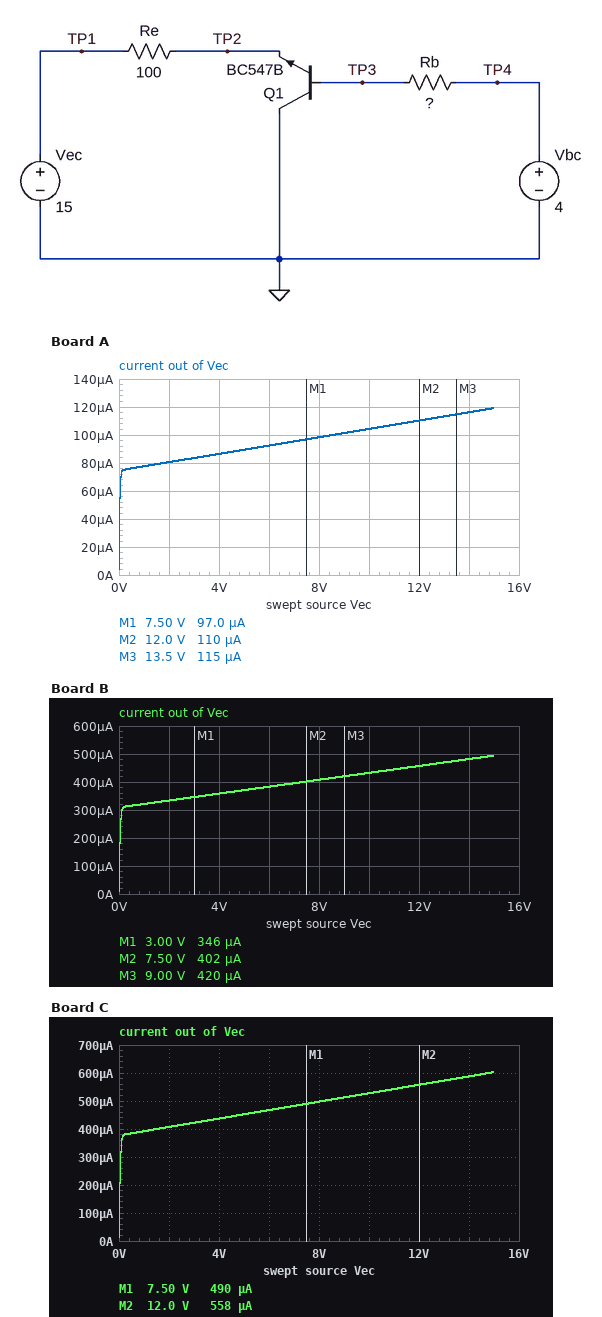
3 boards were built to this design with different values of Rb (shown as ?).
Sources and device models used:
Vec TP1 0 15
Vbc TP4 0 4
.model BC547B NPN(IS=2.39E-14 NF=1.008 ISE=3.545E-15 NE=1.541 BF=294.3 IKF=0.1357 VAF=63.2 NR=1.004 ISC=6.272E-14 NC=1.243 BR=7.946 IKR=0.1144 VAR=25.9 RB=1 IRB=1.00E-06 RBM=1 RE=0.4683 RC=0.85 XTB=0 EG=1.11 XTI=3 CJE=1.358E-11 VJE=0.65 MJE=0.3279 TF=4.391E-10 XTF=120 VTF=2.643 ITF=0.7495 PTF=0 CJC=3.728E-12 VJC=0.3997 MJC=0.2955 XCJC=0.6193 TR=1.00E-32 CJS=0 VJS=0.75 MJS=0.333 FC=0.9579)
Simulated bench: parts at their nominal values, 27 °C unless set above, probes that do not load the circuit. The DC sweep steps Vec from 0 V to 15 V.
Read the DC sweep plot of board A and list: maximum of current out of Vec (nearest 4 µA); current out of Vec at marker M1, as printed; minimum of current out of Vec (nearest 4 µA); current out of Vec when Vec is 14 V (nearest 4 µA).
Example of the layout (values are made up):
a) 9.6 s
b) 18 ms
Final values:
a) 120 µA
b) 97.0 µA
c) 4 µA
d) 116 µA
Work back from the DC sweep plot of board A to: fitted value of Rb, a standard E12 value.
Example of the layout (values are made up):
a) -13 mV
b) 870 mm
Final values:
a) 270 kΩ
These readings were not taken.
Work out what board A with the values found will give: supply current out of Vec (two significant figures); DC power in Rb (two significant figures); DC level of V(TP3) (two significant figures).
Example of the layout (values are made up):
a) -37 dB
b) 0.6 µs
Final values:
a) 120 µA
b) 44 µW
c) 570 mV
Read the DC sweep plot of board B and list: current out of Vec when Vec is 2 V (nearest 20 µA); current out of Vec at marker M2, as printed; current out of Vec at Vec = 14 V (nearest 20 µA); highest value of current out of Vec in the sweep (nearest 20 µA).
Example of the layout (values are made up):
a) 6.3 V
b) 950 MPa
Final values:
a) 340 µA
b) 402 µA
c) 480 µA
d) 500 µA
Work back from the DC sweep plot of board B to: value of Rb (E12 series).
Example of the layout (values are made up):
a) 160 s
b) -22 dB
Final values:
a) 68 kΩ
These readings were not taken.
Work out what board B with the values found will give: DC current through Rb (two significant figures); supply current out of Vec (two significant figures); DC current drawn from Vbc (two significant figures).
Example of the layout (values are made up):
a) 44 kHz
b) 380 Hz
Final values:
a) 50 µA
b) 490 µA
c) 50 µA
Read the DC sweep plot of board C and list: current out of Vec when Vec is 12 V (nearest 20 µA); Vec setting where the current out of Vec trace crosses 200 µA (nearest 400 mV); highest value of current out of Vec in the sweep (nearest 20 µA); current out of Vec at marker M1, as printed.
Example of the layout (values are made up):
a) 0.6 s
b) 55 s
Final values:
a) 560 µA
b) 0 V
c) 600 µA
d) 490 µA
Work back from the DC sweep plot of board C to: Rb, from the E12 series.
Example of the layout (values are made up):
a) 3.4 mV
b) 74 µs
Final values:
a) 56 kΩ
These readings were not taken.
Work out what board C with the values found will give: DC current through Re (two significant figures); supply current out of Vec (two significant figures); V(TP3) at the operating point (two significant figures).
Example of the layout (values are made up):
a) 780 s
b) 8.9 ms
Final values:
a) 600 µA
b) 600 µA
c) 610 mV
